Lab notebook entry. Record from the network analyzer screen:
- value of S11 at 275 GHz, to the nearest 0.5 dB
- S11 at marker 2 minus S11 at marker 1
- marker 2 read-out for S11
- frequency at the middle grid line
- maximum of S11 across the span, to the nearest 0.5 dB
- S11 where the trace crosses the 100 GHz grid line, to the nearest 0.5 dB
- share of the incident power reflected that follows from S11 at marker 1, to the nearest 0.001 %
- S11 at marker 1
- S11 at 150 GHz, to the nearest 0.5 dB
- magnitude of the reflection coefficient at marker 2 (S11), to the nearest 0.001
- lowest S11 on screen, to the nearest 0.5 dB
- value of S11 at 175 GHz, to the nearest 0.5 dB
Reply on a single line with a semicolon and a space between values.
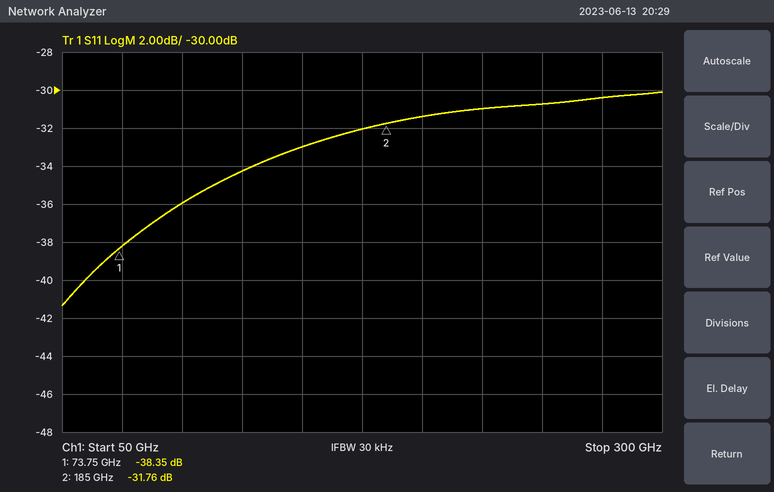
-30.5 dB; 6.59 dB; -31.76 dB; 175 GHz; -30.0 dB; -36.0 dB; 0.015 %; -38.35 dB; -33.0 dB; 0.026; -41.5 dB; -32.0 dB
